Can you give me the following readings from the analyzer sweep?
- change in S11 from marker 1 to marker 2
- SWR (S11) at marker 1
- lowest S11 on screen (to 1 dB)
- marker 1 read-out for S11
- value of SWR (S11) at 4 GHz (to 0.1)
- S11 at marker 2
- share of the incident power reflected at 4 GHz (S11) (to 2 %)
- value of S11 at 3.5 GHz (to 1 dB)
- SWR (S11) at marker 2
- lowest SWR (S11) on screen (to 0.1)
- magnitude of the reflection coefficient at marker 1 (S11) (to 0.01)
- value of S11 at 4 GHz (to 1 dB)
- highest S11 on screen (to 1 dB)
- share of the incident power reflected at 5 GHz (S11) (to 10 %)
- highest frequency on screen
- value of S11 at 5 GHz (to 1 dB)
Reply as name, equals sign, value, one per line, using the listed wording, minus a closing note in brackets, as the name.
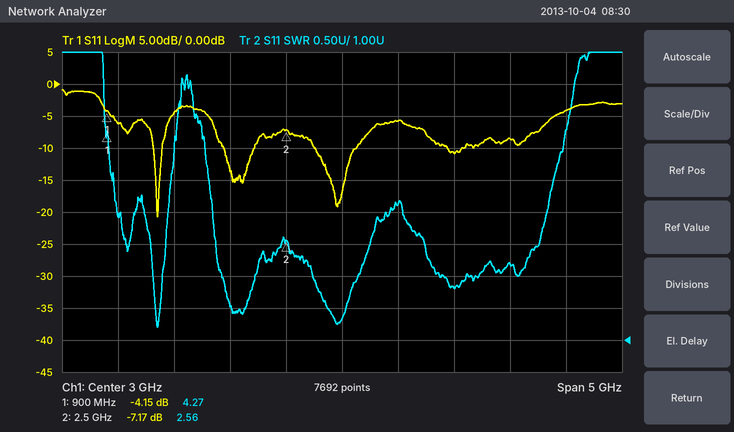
change in S11 from marker 1 to marker 2 = -3.02 dB
SWR (S11) at marker 1 = 4.27
lowest S11 on screen = -21 dB
marker 1 read-out for S11 = -4.15 dB
value of SWR (S11) at 4 GHz = 1.8
S11 at marker 2 = -7.17 dB
share of the incident power reflected at 4 GHz (S11) = 8 %
value of S11 at 3.5 GHz = -6 dB
SWR (S11) at marker 2 = 2.56
lowest SWR (S11) on screen = 1.2
magnitude of the reflection coefficient at marker 1 (S11) = 0.62
value of S11 at 4 GHz = -11 dB
highest S11 on screen = -1 dB
share of the incident power reflected at 5 GHz (S11) = 40 %
highest frequency on screen = 5.5 GHz
value of S11 at 5 GHz = -4 dB
